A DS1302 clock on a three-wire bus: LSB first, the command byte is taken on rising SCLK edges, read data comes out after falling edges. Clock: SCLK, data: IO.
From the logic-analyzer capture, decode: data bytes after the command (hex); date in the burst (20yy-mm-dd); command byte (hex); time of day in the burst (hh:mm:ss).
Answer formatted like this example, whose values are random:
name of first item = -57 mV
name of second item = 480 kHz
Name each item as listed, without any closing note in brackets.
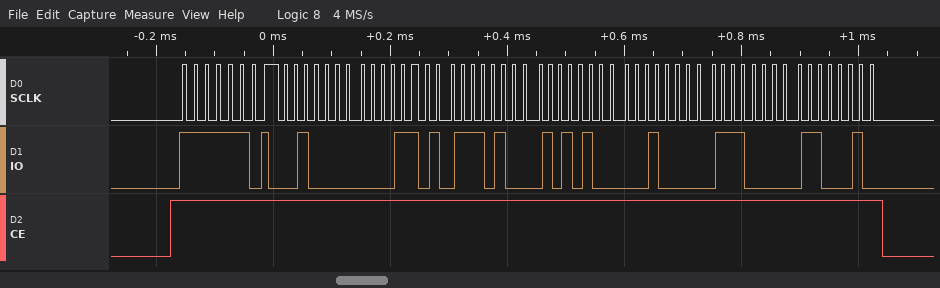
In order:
data bytes after the command = 04 58 17 15 04 07 23
date in the burst = 2023-04-15
command byte = 0xBF
time of day in the burst = 17:58:04
